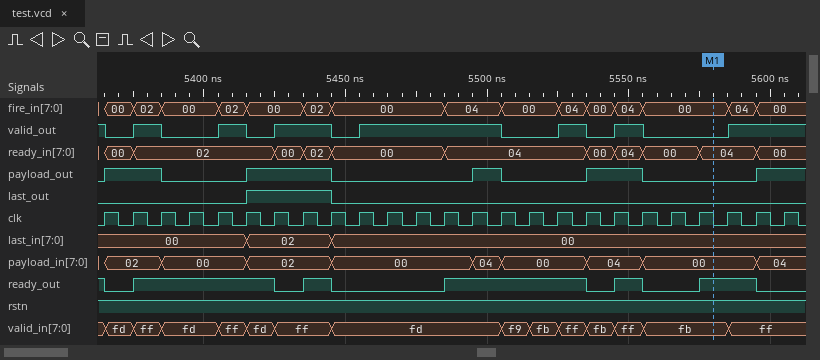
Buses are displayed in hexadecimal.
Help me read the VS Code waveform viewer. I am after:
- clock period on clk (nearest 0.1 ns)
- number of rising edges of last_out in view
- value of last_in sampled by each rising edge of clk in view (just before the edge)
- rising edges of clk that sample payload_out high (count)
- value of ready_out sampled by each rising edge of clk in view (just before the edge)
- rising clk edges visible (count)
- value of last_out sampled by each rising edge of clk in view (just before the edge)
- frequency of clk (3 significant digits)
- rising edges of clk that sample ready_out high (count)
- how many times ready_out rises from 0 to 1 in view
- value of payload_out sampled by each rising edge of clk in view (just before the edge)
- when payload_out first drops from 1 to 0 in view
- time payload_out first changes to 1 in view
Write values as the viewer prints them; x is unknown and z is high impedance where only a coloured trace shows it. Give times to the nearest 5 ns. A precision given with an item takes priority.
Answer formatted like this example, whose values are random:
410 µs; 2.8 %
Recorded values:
10 ns; 1; 00, 00, 00, 00, 00, 00, 02, 02, 02, 00, 00, 00, 00, 00, 00, 00, 00, 00, 00, 00, 00, 00, 00, 00, 00; 9; 1 0 1 1 1 1 1 0 1 0 0 0 0 1 1 1 1 1 0 1 0 0 1 1 0; 25; 0 0 0 0 0 0 1 1 1 0 0 0 0 0 0 0 0 0 0 0 0 0 0 0 0; 100 MHz; 15; 5; 0 1 1 0 0 0 1 1 1 0 0 0 0 0 1 0 0 0 1 1 0 0 0 0 1; 5385 ns; 5365 ns
